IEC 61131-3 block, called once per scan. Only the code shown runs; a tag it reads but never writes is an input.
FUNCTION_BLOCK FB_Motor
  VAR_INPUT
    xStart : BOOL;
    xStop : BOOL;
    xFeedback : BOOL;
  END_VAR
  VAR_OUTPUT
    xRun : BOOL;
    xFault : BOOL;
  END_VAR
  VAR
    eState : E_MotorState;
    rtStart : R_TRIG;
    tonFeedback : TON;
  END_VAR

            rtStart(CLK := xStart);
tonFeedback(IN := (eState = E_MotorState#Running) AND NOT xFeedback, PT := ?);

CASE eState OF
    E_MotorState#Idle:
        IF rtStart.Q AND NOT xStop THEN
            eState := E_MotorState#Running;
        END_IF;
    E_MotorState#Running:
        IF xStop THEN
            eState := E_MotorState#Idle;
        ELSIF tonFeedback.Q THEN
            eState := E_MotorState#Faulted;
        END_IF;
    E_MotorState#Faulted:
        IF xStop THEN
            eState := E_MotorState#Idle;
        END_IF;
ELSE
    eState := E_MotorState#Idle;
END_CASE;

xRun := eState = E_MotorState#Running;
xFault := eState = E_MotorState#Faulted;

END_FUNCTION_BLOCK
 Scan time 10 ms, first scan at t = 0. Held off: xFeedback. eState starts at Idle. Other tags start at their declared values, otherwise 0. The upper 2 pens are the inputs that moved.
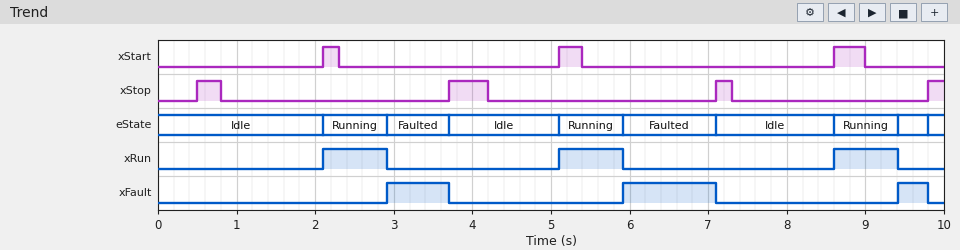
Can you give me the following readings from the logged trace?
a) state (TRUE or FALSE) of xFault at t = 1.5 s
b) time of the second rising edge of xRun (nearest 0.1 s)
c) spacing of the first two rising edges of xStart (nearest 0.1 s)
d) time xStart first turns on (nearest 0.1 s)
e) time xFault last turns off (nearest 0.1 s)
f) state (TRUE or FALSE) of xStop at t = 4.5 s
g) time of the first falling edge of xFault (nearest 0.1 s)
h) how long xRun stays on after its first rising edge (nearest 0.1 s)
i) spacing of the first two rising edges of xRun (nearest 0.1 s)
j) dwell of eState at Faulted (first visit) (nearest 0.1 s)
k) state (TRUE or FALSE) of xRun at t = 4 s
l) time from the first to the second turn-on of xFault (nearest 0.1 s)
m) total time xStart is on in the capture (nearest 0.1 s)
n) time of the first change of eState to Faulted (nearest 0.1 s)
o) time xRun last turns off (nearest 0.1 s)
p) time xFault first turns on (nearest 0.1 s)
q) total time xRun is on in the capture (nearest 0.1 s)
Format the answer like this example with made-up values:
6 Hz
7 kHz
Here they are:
FALSE
5.1 s
3.0 s
2.1 s
9.8 s
FALSE
3.7 s
0.8 s
3.0 s
0.8 s
FALSE
3.0 s
0.9 s
2.9 s
9.4 s
2.9 s
2.4 s
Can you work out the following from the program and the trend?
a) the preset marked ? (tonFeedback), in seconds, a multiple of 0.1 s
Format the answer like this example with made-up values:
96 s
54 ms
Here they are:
0.8 s
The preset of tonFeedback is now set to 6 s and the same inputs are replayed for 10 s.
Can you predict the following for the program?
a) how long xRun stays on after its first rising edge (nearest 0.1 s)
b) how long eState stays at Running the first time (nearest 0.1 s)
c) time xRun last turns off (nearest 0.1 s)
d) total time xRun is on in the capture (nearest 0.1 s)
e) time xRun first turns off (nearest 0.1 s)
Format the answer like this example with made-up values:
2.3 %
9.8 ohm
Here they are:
1.6 s
1.6 s
9.8 s
4.8 s
3.7 s
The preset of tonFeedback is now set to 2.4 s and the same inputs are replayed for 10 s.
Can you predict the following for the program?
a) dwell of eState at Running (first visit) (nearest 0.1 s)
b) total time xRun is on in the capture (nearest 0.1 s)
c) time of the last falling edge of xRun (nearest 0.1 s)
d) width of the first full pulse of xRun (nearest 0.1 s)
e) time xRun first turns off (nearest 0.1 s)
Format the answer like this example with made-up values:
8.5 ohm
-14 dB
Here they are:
1.6 s
4.8 s
9.8 s
1.6 s
3.7 s
